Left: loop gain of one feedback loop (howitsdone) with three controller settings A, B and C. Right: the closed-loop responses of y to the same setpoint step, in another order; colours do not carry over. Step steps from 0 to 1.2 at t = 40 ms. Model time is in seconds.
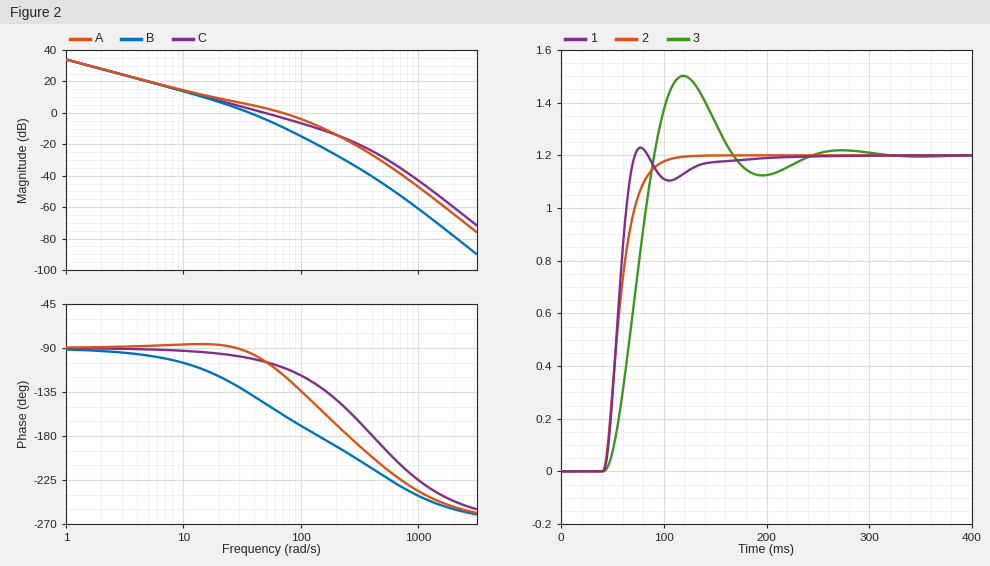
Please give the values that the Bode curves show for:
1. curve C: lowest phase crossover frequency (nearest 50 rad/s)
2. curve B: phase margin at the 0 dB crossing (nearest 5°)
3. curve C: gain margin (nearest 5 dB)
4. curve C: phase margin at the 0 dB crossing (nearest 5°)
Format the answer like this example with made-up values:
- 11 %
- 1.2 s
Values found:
- 400 rad/s
- 45°
- 25 dB
- 75°
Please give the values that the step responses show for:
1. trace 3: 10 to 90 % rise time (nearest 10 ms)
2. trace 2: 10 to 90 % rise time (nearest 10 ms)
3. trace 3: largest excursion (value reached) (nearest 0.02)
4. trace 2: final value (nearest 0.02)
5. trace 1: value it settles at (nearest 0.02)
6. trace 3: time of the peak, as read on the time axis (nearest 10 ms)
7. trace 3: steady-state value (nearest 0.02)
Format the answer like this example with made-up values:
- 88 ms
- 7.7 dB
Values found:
- 30 ms
- 30 ms
- 1.50
- 1.20
- 1.20
- 120 ms
- 1.20
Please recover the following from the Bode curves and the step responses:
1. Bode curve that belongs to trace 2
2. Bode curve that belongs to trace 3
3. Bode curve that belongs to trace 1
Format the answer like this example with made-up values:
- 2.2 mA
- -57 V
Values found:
- C
- B
- A
